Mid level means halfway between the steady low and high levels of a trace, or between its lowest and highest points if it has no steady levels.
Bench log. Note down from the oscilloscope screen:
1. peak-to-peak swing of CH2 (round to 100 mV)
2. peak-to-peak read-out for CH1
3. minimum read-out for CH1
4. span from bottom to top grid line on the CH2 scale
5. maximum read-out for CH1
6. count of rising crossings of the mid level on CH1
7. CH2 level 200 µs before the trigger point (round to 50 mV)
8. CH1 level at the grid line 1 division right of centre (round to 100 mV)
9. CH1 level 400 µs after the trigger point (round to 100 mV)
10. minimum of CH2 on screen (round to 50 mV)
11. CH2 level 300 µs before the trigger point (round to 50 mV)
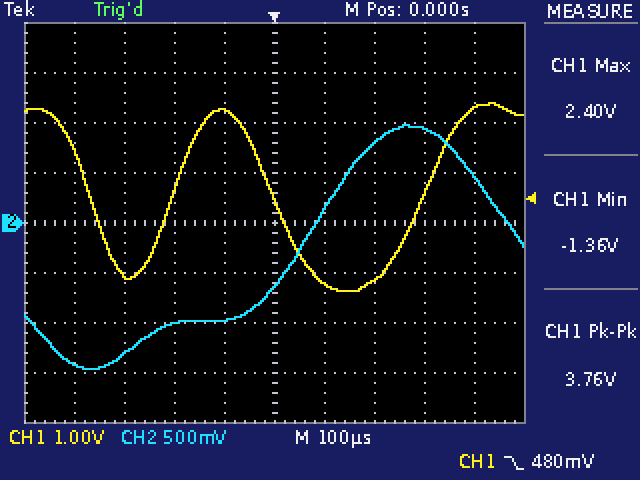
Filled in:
2.40 V
3.76 V
-1.36 V
4 V
2.40 V
2
-1.00 V
-1.2 V
2.3 V
-1.45 V
-1.30 V
